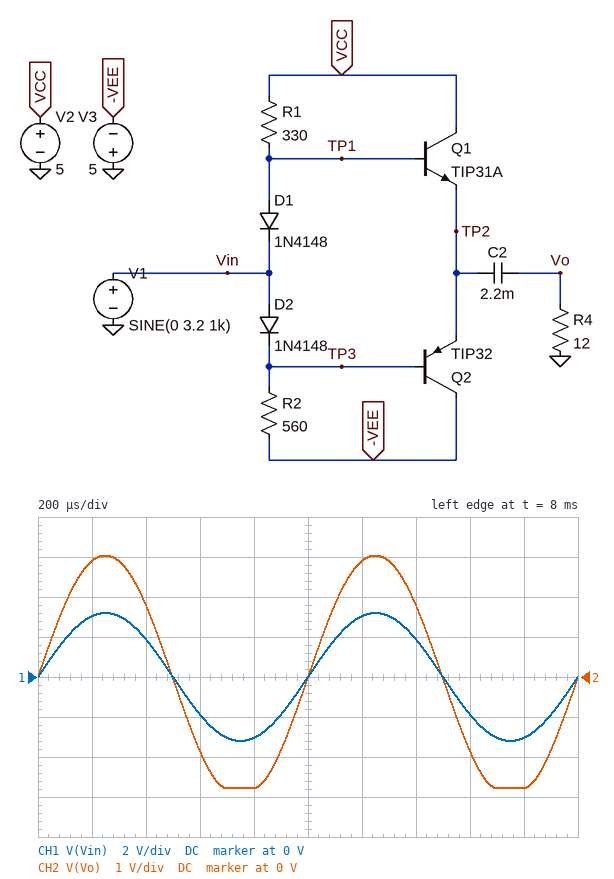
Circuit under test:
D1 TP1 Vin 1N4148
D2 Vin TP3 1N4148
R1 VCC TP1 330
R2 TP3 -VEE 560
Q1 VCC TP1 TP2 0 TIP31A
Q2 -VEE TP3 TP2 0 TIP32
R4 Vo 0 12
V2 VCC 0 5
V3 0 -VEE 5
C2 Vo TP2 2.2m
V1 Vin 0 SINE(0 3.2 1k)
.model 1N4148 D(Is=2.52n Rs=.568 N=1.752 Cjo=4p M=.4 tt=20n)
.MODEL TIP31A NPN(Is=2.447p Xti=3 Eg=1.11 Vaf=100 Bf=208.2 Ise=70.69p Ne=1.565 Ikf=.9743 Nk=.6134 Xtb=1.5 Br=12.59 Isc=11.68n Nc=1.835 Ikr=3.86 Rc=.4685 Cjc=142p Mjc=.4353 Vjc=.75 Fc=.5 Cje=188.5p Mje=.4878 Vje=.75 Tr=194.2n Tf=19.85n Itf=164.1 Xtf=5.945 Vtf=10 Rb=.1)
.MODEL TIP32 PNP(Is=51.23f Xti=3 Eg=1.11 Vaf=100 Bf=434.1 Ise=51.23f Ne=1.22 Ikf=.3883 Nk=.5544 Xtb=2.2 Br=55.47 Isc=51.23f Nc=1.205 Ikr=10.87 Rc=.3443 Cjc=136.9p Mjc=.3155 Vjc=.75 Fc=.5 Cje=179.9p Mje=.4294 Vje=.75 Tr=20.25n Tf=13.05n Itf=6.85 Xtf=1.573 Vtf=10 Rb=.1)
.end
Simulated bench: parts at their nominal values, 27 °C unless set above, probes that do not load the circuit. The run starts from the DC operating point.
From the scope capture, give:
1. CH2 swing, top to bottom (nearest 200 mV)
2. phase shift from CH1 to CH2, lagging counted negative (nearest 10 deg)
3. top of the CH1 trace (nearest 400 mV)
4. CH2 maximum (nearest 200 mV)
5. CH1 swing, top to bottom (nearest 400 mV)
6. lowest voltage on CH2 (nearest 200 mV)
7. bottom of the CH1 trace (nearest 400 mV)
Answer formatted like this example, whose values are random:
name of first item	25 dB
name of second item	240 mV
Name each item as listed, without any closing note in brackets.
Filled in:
CH2 swing, top to bottom	5.8 V
phase shift from CH1 to CH2, lagging counted negative	0 deg
top of the CH1 trace	3.2 V
CH2 maximum	3.0 V
CH1 swing, top to bottom	6.4 V
lowest voltage on CH2	-2.8 V
bottom of the CH1 trace	-3.2 V
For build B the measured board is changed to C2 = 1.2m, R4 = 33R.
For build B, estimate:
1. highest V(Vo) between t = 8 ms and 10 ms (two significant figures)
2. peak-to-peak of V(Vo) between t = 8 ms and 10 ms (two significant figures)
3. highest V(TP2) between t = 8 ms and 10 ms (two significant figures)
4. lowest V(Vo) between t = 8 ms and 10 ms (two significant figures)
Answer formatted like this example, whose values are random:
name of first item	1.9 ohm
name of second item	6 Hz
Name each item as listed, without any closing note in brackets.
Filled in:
highest V(Vo) between t = 8 ms and 10 ms	3.1 V
peak-to-peak of V(Vo) between t = 8 ms and 10 ms	6.2 V
highest V(TP2) between t = 8 ms and 10 ms	3.2 V
lowest V(Vo) between t = 8 ms and 10 ms	-3.1 V
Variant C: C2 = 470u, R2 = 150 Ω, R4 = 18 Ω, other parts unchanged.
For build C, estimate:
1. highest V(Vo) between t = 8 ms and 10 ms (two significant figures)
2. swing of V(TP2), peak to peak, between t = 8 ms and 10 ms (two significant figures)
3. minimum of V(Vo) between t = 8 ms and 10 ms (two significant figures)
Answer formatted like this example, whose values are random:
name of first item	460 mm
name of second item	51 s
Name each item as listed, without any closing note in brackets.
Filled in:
highest V(Vo) between t = 8 ms and 10 ms	3.1 V
swing of V(TP2), peak to peak, between t = 8 ms and 10 ms	6.2 V
minimum of V(Vo) between t = 8 ms and 10 ms	-3.1 V
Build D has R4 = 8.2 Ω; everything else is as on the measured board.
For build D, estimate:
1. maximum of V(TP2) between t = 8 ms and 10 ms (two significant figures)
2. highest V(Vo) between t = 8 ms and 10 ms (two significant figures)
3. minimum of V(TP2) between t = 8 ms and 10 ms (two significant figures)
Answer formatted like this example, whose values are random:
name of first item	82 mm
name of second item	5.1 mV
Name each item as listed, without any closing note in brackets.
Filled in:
maximum of V(TP2) between t = 8 ms and 10 ms	3.0 V
highest V(Vo) between t = 8 ms and 10 ms	2.9 V
minimum of V(TP2) between t = 8 ms and 10 ms	-2.2 V
